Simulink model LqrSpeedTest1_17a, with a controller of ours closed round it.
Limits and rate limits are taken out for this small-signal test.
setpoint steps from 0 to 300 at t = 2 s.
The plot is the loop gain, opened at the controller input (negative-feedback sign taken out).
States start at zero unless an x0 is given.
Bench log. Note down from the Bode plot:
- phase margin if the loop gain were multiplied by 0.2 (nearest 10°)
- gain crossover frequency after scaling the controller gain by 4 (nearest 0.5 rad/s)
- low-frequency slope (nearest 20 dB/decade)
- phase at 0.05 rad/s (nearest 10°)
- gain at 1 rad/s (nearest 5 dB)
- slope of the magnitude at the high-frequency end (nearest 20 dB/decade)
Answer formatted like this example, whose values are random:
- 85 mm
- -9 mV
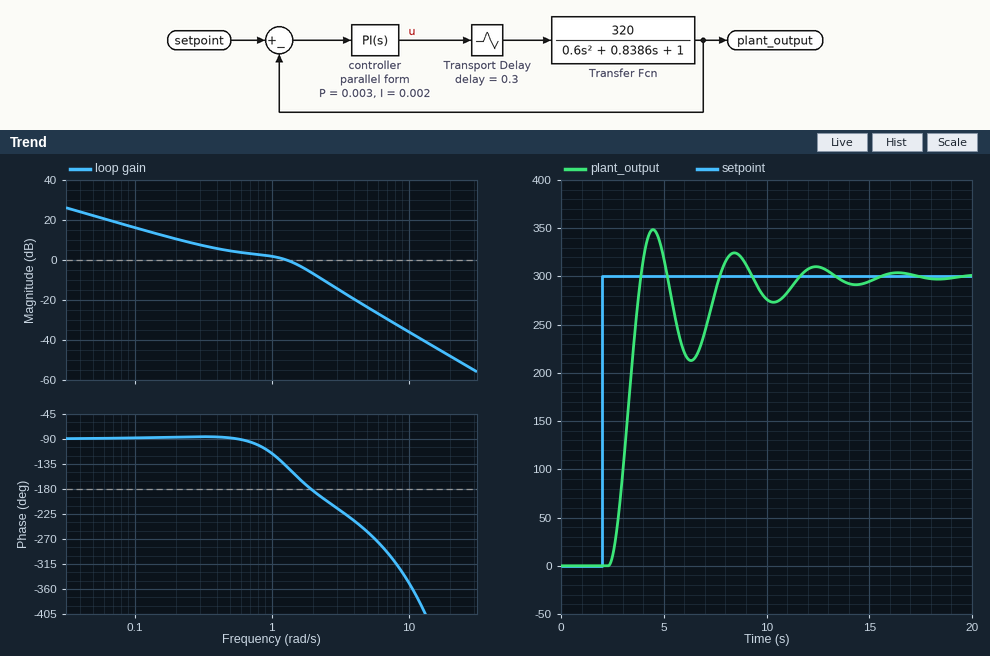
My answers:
- 90°
- 2.5 rad/s
- -20 dB/decade
- -90°
- 0 dB
- -40 dB/decade
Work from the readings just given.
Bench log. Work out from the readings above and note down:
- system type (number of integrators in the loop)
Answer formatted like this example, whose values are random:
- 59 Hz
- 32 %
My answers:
- 1
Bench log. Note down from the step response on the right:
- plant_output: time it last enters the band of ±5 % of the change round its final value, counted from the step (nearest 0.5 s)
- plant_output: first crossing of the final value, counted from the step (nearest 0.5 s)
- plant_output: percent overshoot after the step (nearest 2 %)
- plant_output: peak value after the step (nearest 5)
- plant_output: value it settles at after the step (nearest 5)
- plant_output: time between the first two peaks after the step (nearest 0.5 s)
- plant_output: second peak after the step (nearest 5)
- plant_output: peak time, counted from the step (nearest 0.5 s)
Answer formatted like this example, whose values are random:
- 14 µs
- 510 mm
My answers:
- 9.0 s
- 2.0 s
- 16 %
- 350
- 300
- 4.0 s
- 325
- 2.5 s
